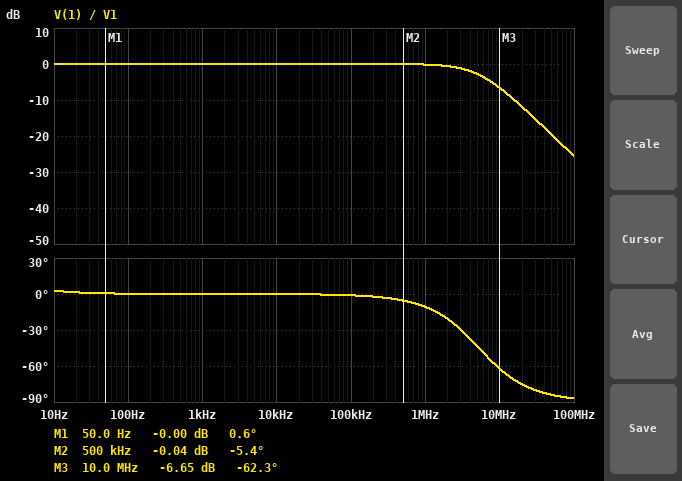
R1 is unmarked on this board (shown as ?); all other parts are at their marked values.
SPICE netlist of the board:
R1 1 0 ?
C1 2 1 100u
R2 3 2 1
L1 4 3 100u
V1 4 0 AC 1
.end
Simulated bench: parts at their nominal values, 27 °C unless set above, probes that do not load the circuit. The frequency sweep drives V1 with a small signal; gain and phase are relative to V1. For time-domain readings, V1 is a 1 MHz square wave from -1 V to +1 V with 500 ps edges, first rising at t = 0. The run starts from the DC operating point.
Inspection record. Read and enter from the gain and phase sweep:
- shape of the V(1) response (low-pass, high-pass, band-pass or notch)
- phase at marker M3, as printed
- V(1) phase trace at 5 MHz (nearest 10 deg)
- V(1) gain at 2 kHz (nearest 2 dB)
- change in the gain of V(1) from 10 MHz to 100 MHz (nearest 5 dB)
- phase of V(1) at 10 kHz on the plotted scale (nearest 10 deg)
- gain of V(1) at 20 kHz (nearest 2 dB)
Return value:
low-pass
-62.3 deg
-40 deg
0 dB
-20 dB
0 deg
0 dB
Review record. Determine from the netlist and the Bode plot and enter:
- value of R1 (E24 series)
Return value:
3.3 kΩ
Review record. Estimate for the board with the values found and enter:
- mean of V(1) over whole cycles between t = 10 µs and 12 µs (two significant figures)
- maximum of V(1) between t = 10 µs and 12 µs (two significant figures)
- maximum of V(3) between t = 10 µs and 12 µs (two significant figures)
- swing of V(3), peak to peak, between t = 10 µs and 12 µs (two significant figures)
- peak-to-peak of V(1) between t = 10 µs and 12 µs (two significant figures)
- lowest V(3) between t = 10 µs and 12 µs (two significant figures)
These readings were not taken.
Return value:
1.0 V
2.0 V
1.0 V
2.0 V
2.0 V
-1.0 V
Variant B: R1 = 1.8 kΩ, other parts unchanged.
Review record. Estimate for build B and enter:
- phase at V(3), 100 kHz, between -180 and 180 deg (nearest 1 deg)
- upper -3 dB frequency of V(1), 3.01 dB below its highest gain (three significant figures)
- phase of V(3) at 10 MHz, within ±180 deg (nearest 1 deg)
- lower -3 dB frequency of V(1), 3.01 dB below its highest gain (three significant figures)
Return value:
-2 deg
2.87 MHz
-74 deg
884 mHz
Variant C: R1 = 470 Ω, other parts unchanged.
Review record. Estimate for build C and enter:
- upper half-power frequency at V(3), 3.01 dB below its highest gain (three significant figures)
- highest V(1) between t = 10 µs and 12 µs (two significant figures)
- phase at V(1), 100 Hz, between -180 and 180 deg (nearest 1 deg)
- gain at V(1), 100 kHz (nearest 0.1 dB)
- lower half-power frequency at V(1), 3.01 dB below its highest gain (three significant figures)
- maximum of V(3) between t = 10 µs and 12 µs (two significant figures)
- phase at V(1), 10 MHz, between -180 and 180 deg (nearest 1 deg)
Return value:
750 kHz
1.8 V
2 deg
-0.1 dB
3.38 Hz
830 mV
-86 deg
